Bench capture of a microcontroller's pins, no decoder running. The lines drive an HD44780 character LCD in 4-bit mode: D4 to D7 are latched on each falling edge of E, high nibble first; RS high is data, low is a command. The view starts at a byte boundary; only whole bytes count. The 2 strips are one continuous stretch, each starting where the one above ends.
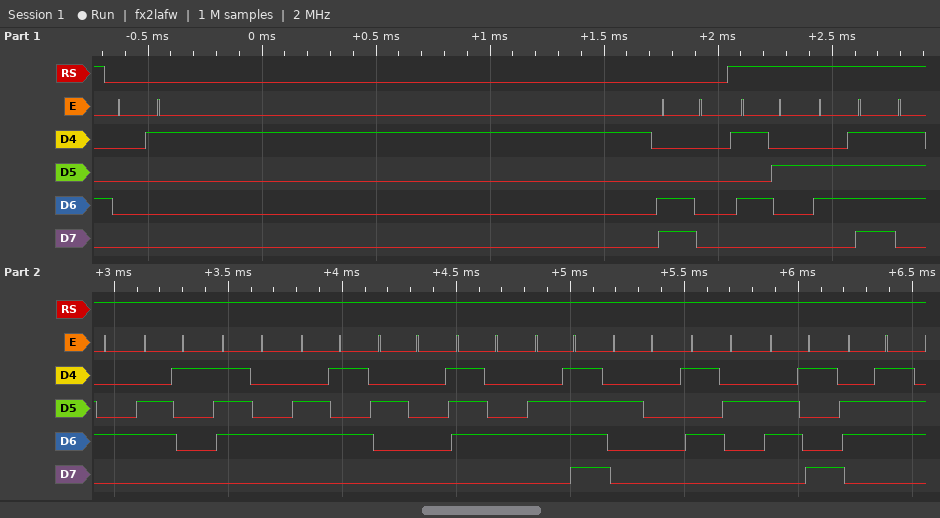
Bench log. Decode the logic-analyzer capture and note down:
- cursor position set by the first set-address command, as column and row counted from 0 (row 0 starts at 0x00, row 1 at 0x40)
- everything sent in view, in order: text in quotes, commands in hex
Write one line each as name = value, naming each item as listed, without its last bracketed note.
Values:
cursor position set by the first set-address command, as column and row counted from 0 = column 0, row 1
everything sent in view, in order: text in quotes, commands in hex = 0x01 0xC0 "Rotate to Rig"
